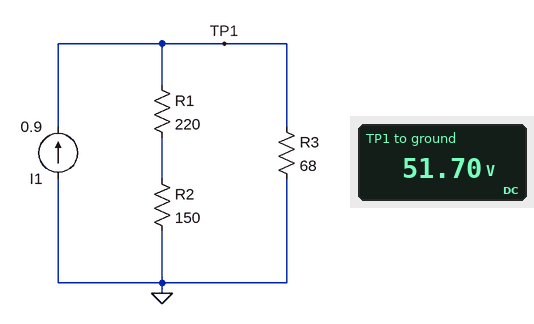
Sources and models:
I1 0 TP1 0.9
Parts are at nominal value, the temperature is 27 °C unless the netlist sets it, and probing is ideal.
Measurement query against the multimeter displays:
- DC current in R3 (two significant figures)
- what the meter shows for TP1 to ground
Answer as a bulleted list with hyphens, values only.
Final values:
- 760 mA
- 51.70 V
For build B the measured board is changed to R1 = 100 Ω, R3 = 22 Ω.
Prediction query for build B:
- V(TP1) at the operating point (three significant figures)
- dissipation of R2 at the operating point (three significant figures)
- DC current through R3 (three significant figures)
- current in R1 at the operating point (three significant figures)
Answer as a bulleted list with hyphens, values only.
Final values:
- 18.2 V
- 795 mW
- 827 mA
- 72.8 mA
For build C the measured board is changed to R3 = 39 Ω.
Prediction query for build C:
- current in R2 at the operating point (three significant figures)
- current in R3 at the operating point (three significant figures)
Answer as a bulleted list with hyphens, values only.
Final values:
- 85.8 mA
- 814 mA
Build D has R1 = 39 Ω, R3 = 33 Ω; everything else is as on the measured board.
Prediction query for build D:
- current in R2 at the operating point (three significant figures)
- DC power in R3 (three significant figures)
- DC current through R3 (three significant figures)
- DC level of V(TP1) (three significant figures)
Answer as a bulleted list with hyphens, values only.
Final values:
- 134 mA
- 19.4 W
- 766 mA
- 25.3 V
